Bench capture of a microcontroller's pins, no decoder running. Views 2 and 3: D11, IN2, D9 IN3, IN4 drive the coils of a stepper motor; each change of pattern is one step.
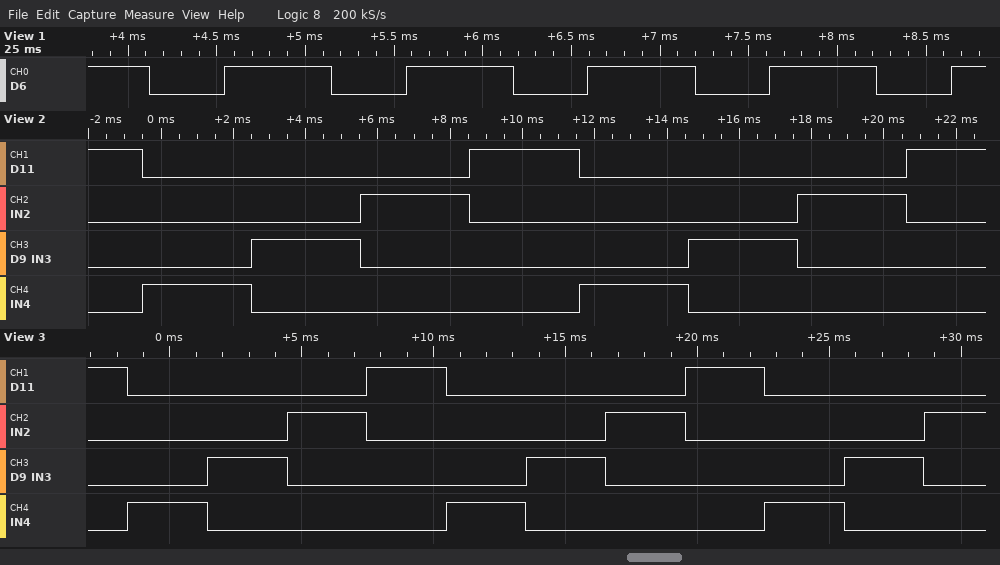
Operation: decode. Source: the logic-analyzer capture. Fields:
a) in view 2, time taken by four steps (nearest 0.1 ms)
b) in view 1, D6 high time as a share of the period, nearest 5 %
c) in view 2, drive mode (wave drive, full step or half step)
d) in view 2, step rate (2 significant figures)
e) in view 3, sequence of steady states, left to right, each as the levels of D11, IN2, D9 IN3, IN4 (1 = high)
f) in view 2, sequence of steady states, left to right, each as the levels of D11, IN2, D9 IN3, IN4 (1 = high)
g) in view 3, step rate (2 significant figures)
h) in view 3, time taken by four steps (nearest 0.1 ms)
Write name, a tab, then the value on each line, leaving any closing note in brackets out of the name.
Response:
in view 2, time taken by four steps	12.1 ms
in view 1, D6 high time as a share of the period, nearest 5 %	60 %
in view 2, drive mode	wave drive
in view 2, step rate	330 steps/s
in view 3, sequence of steady states, left to right, each as the levels of D11, IN2, D9 IN3, IN4	1000 0001 0010 0100 1000 0001 0010 0100 1000 0001 0010 0100
in view 2, sequence of steady states, left to right, each as the levels of D11, IN2, D9 IN3, IN4	1000 0001 0010 0100 1000 0001 0010 0100 1000
in view 3, step rate	330 steps/s
in view 3, time taken by four steps	12.1 ms
